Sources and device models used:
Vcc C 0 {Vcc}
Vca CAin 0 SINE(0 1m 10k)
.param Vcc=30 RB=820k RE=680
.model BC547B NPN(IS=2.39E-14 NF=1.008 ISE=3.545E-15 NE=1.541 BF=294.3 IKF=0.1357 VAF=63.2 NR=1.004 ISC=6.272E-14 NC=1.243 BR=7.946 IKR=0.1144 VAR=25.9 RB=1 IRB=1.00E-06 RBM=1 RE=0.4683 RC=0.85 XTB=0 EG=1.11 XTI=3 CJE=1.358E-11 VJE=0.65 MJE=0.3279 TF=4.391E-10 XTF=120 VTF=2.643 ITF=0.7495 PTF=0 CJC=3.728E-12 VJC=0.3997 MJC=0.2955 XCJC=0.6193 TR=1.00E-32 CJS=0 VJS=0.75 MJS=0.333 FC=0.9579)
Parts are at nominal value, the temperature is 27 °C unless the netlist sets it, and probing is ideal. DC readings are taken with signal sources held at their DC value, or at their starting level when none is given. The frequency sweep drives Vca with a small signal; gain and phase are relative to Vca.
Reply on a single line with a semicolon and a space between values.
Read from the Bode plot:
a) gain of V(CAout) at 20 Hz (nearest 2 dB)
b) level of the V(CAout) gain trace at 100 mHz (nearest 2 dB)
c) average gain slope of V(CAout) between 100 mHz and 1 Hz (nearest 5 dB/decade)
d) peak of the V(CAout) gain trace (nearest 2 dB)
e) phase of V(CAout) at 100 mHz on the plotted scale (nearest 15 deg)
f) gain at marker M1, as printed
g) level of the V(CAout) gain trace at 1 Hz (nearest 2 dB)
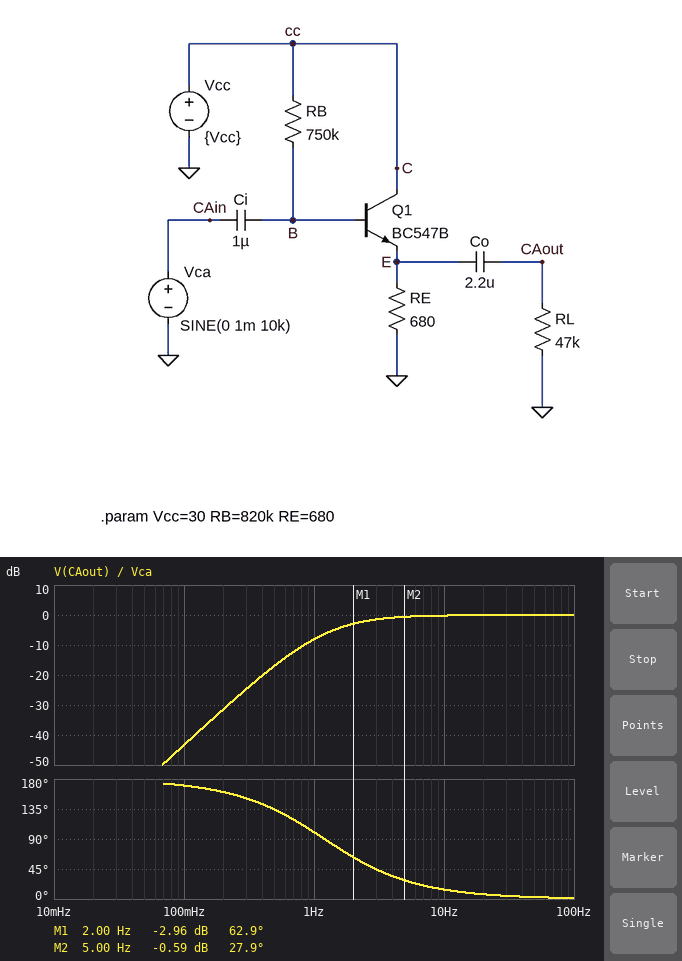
0 dB; -44 dB; 35 dB/decade; 0 dB; 165 deg; -2.96 dB; -8 dB
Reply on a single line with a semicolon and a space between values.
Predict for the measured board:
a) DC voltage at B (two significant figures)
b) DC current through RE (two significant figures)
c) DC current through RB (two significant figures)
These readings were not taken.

8.0 V; 11 mA; 29 µA
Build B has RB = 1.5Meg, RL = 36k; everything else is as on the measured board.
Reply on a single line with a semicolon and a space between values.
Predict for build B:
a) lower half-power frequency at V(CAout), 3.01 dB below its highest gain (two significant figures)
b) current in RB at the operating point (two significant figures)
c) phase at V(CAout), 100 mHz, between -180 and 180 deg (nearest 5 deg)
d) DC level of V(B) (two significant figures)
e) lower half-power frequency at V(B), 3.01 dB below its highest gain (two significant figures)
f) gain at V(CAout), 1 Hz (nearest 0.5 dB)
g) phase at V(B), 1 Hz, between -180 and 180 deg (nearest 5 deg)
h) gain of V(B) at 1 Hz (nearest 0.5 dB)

2.3 Hz; 17 µA; 170 deg; 5.1 V; 760 mHz; -9.0 dB; 35 deg; -2.0 dB
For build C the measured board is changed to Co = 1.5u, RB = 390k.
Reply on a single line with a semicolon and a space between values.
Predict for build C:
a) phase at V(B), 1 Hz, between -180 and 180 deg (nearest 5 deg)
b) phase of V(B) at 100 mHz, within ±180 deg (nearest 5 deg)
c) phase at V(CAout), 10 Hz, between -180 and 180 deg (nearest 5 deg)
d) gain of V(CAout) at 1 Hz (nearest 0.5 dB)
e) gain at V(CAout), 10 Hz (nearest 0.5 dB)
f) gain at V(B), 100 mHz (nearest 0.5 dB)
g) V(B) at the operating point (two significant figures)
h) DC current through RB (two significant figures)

50 deg; 85 deg; 20 deg; -12.0 dB; -0.5 dB; -22.0 dB; 12 V; 47 µA
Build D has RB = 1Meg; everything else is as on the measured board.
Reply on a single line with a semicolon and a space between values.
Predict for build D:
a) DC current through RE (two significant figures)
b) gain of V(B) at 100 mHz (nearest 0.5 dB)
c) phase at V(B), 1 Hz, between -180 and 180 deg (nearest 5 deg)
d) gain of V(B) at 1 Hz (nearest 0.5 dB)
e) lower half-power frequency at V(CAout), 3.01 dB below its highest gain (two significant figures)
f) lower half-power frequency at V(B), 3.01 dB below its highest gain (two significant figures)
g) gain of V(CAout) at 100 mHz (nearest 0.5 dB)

8.8 mA; -18.5 dB; 40 deg; -2.5 dB; 1.9 Hz; 860 mHz; -42.5 dB
